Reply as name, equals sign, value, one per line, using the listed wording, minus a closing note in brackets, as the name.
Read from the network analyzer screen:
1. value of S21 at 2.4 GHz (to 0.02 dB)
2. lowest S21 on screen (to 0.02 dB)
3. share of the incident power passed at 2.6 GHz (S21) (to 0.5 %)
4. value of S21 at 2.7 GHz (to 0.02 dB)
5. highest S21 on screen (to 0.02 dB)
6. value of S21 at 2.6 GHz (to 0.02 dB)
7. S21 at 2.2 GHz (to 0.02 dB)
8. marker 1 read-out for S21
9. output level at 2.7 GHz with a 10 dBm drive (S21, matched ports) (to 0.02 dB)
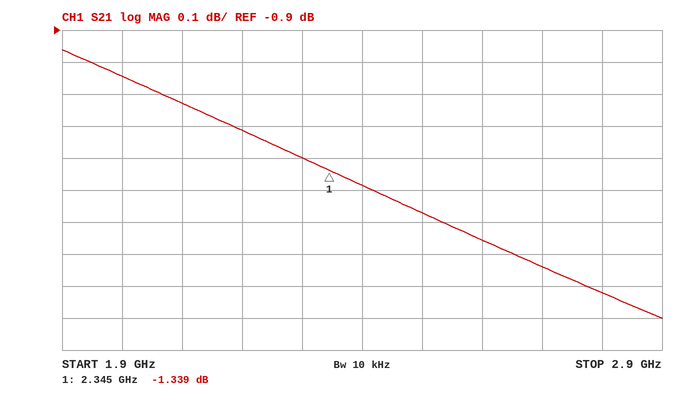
value of S21 at 2.4 GHz = -1.38 dB
lowest S21 on screen = -1.80 dB
share of the incident power passed at 2.6 GHz (S21) = 70.0 %
value of S21 at 2.7 GHz = -1.64 dB
highest S21 on screen = -0.96 dB
value of S21 at 2.6 GHz = -1.56 dB
S21 at 2.2 GHz = -1.22 dB
marker 1 read-out for S21 = -1.339 dB
output level at 2.7 GHz with a 10 dBm drive (S21, matched ports) = 8.36 dBm
